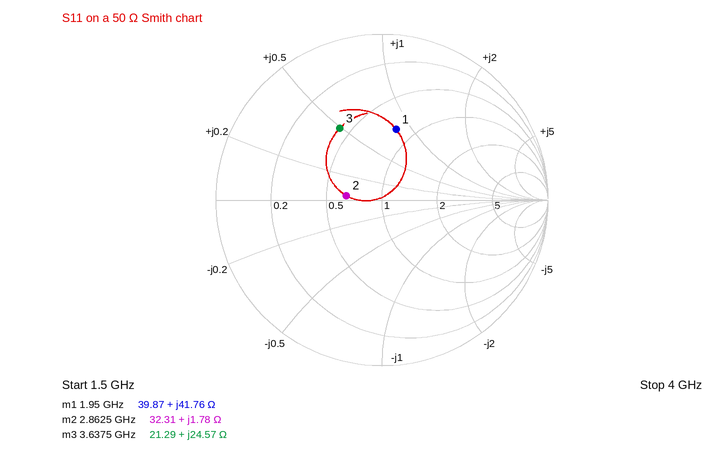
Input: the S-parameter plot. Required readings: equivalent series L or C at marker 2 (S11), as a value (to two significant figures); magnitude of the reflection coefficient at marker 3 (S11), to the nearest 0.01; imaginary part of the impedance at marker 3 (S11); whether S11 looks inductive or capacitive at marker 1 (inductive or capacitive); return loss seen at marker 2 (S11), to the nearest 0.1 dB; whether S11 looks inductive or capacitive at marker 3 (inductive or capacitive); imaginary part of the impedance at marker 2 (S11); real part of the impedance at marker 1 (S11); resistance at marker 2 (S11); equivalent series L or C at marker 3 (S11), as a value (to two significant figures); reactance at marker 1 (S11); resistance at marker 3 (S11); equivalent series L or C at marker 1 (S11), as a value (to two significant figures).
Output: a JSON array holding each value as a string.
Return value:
["99 pH", "0.50", "+24.57 Ω", "inductive", "13.3 dB", "inductive", "+1.78 Ω", "39.87 Ω", "32.31 Ω", "1.1 nH", "+41.76 Ω", "21.29 Ω", "3.4 nH"]
